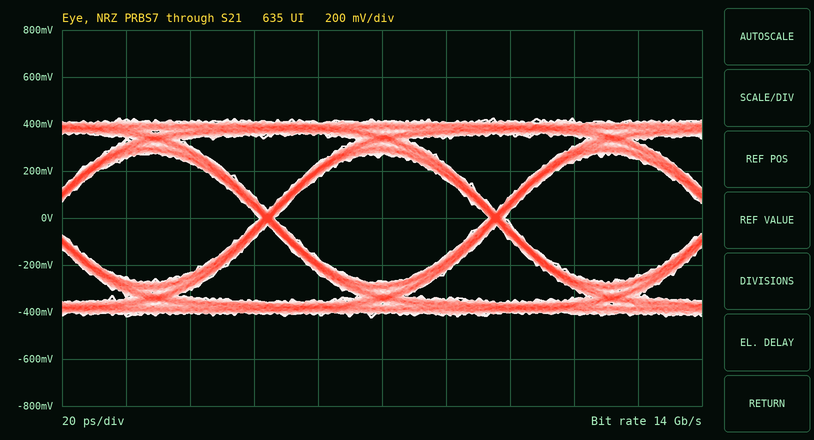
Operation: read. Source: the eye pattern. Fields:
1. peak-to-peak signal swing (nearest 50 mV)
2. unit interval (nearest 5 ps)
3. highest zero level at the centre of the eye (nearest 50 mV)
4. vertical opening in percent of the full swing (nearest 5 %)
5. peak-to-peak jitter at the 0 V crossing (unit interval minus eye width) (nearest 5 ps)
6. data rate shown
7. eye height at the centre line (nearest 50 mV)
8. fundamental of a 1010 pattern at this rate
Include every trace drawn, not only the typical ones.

850 mV
70 ps
-250 mV
65 %
5 ps
14 Gb/s
550 mV
7 GHz
